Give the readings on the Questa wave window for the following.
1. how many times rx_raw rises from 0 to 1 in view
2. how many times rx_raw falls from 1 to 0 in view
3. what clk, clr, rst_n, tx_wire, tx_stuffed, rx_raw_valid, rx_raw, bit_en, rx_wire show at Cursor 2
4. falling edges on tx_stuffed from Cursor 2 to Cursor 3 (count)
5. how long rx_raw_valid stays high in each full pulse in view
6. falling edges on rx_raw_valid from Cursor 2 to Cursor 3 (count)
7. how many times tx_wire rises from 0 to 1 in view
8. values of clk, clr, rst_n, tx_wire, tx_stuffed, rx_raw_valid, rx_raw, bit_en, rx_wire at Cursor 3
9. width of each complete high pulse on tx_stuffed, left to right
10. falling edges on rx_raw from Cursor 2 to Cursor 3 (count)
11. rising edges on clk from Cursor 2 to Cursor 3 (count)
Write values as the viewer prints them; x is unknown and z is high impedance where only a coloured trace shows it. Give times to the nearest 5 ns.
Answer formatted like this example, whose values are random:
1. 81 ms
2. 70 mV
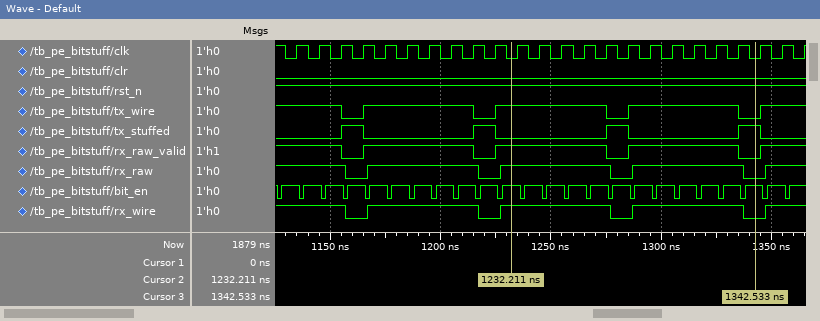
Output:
1. 4
2. 4
3. clk=0, clr=0, rst_n=1, tx_wire=1, tx_stuffed=0, rx_raw_valid=1, rx_raw=1, bit_en=1, rx_wire=1
4. 1
5. 50 ns, 50 ns, 50 ns
6. 2
7. 4
8. clk=0, clr=0, rst_n=1, tx_wire=0, tx_stuffed=1, rx_raw_valid=0, rx_raw=0, bit_en=1, rx_wire=0
9. 10 ns, 10 ns, 10 ns, 10 ns
10. 2
11. 11
